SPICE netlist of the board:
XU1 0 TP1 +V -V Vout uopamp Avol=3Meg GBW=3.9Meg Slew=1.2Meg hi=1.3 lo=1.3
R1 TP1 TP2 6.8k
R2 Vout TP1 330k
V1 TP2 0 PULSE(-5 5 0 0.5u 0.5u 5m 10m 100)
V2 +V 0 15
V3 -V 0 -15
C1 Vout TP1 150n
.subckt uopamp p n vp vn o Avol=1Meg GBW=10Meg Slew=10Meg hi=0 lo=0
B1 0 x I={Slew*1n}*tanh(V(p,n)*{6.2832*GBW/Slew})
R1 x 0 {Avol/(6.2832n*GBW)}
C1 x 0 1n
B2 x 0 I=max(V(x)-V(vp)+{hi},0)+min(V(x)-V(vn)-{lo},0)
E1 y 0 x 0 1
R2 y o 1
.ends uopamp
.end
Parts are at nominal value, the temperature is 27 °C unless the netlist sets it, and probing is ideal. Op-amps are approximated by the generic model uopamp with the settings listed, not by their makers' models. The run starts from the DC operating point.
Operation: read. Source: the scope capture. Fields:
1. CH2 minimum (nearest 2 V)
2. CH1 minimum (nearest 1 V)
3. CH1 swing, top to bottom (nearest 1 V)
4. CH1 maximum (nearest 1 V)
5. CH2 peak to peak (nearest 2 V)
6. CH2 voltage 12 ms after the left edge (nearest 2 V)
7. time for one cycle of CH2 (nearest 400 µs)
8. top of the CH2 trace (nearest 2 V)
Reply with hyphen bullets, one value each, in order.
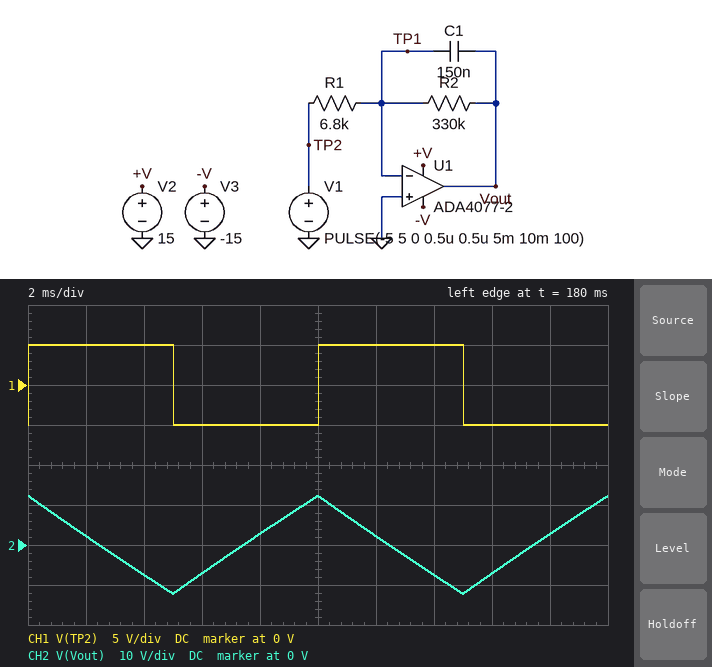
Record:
- -12 V
- -5 V
- 10 V
- 5 V
- 24 V
- 2 V
- 10.0 ms
- 12 V
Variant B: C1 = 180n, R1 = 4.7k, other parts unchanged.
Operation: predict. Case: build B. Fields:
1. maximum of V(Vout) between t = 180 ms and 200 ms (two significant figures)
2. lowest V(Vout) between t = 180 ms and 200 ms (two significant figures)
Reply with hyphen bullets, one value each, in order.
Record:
- 14 V
- -14 V
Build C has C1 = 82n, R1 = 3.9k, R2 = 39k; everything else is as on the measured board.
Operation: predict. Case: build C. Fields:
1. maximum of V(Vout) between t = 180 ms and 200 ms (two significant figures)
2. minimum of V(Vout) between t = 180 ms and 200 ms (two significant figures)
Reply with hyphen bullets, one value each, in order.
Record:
- 14 V
- -14 V
